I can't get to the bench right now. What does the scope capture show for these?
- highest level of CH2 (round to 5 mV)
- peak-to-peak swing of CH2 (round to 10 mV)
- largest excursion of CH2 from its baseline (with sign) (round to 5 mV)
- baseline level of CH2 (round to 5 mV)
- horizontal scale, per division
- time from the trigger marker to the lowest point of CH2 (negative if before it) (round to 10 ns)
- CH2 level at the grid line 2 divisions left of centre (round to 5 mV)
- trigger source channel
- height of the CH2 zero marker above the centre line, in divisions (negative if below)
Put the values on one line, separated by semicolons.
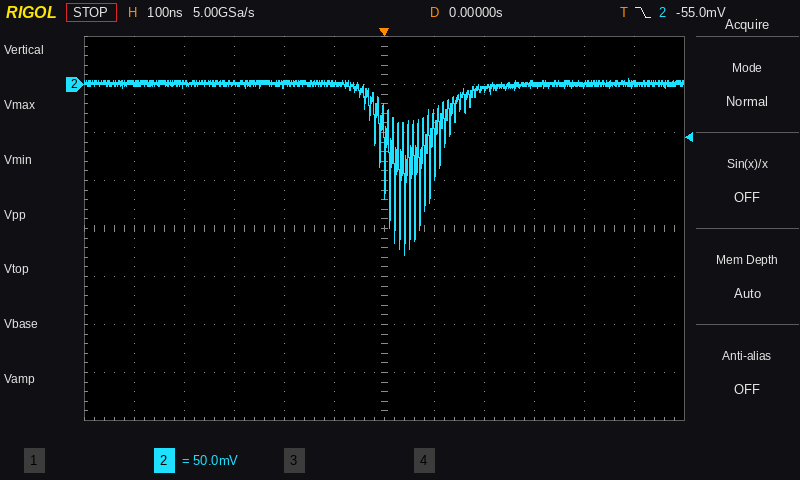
5 mV; 180 mV; -180 mV; 0 mV; 100 ns; +40 ns; 0 mV; CH2; +3.0 div
